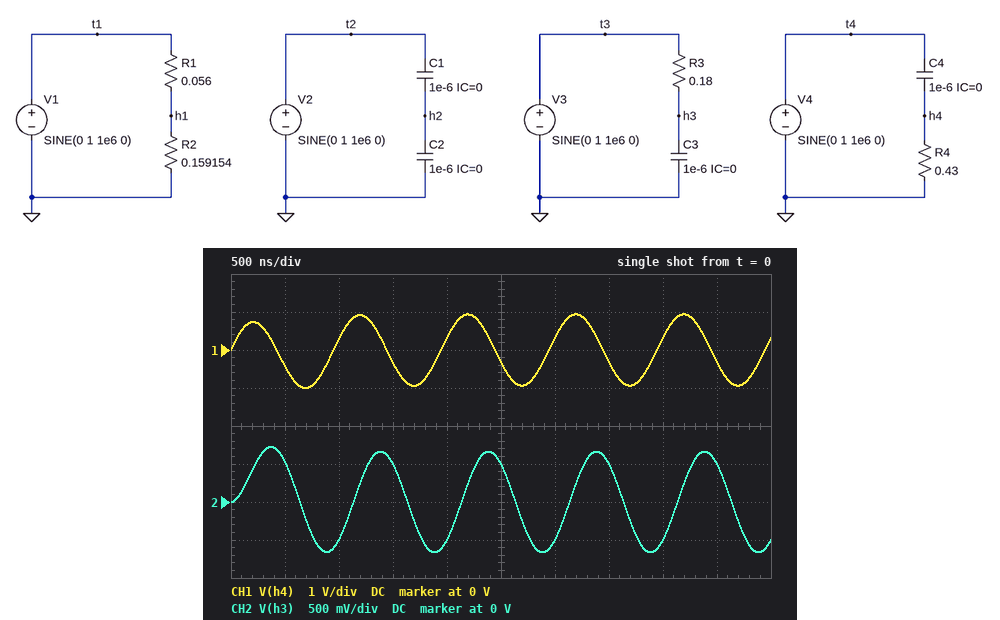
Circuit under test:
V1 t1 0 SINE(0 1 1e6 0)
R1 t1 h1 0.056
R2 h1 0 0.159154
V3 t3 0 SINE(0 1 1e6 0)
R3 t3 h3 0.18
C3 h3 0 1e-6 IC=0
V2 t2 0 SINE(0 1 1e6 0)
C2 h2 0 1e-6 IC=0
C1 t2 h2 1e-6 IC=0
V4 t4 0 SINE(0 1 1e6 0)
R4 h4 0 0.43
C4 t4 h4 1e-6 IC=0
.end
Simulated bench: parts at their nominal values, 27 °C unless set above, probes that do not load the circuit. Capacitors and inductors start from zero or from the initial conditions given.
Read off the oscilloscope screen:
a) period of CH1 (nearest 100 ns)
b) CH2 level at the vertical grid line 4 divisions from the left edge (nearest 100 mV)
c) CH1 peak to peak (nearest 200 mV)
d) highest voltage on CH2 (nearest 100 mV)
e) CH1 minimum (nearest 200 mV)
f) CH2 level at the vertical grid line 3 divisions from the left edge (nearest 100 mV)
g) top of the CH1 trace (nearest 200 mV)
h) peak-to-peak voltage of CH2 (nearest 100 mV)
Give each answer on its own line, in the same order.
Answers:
1.0 µs
-500 mV
2.0 V
700 mV
-1.0 V
500 mV
1.0 V
1.4 V
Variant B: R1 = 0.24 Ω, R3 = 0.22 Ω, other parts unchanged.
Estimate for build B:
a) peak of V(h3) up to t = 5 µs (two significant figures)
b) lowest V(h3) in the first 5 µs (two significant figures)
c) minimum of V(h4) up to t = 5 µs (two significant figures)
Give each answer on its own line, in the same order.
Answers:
670 mV
-590 mV
-1.0 V
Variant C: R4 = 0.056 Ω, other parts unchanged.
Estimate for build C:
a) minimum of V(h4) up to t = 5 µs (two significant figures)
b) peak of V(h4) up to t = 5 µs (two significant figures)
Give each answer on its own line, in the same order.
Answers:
-330 mV
330 mV
